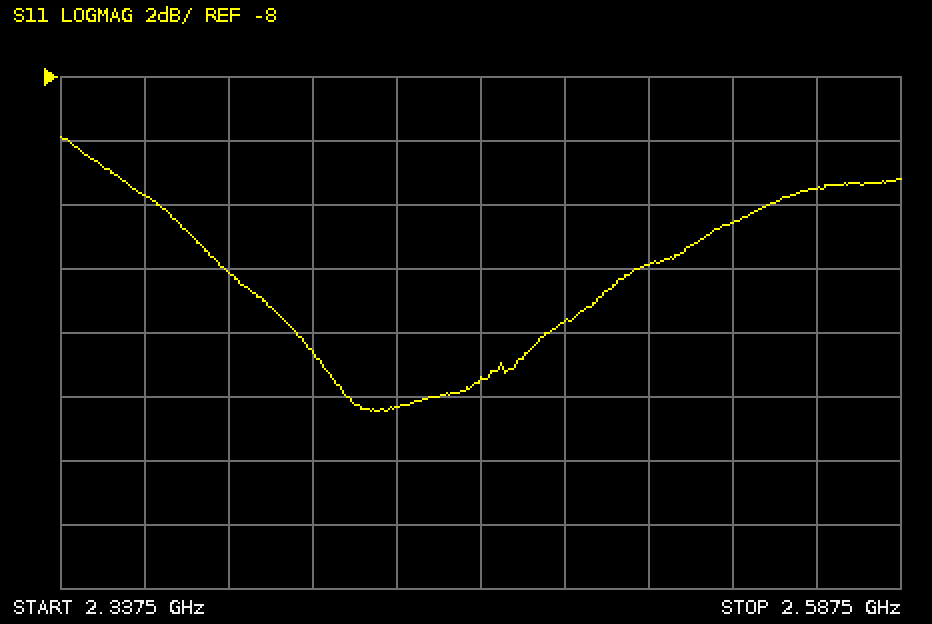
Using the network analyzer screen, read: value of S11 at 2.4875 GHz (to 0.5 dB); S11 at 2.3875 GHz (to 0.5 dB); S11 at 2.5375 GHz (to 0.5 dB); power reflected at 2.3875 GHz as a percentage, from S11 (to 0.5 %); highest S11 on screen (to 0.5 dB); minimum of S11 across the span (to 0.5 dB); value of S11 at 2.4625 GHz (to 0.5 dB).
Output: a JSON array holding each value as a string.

["-15.5 dB", "-14.0 dB", "-12.5 dB", "4.0 %", "-10.0 dB", "-18.5 dB", "-17.5 dB"]
